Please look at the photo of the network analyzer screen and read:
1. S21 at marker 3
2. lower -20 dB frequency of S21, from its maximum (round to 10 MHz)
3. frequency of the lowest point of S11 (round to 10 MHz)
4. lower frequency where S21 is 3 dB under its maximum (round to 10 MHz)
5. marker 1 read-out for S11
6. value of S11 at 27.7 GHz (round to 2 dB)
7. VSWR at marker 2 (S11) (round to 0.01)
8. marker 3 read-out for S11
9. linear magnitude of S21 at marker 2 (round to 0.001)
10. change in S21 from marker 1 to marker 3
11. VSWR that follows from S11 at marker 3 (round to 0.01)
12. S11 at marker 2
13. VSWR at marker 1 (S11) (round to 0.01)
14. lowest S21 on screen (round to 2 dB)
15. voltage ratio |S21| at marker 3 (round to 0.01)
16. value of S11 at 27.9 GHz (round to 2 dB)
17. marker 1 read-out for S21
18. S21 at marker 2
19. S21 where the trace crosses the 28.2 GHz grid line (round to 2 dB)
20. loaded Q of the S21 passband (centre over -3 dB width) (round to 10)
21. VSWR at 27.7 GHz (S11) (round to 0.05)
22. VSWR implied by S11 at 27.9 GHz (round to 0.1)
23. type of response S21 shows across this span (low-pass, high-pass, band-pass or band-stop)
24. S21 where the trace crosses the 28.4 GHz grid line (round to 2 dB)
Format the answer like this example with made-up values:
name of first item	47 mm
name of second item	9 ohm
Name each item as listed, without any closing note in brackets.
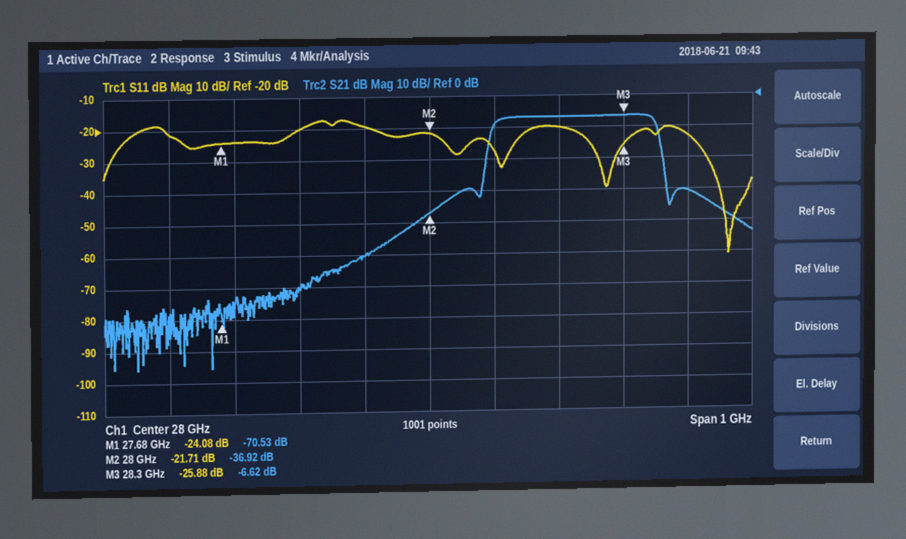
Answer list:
S21 at marker 3	-6.62 dB
lower -20 dB frequency of S21, from its maximum	28.08 GHz
frequency of the lowest point of S11	28.46 GHz
lower frequency where S21 is 3 dB under its maximum	28.10 GHz
marker 1 read-out for S11	-24.08 dB
value of S11 at 27.7 GHz	-24 dB
VSWR at marker 2 (S11)	1.18
marker 3 read-out for S11	-25.88 dB
linear magnitude of S21 at marker 2	0.014
change in S21 from marker 1 to marker 3	63.91 dB
VSWR that follows from S11 at marker 3	1.11
S11 at marker 2	-21.71 dB
VSWR at marker 1 (S11)	1.13
lowest S21 on screen	-86 dB
voltage ratio |S21| at marker 3	0.47
value of S11 at 27.9 GHz	-20 dB
marker 1 read-out for S21	-70.53 dB
S21 at marker 2	-36.92 dB
S21 where the trace crosses the 28.2 GHz grid line	-6 dB
loaded Q of the S21 passband (centre over -3 dB width)	110
VSWR at 27.7 GHz (S11)	1.15
VSWR implied by S11 at 27.9 GHz	1.2
type of response S21 shows across this span	band-pass
S21 where the trace crosses the 28.4 GHz grid line	-30 dB
